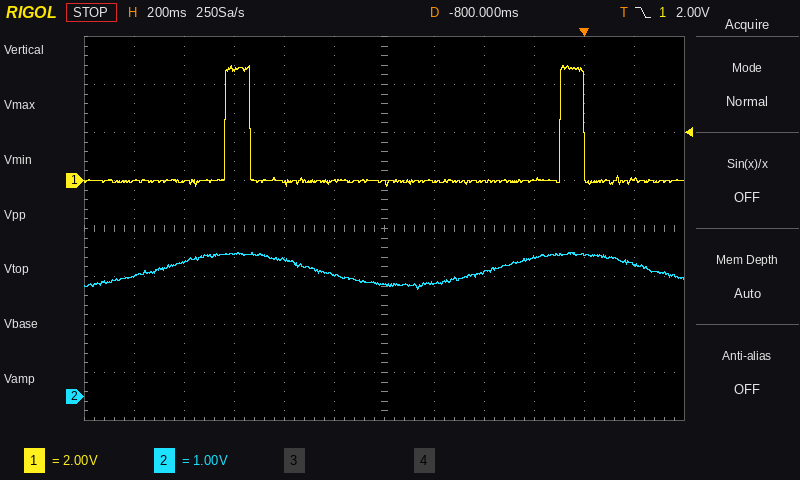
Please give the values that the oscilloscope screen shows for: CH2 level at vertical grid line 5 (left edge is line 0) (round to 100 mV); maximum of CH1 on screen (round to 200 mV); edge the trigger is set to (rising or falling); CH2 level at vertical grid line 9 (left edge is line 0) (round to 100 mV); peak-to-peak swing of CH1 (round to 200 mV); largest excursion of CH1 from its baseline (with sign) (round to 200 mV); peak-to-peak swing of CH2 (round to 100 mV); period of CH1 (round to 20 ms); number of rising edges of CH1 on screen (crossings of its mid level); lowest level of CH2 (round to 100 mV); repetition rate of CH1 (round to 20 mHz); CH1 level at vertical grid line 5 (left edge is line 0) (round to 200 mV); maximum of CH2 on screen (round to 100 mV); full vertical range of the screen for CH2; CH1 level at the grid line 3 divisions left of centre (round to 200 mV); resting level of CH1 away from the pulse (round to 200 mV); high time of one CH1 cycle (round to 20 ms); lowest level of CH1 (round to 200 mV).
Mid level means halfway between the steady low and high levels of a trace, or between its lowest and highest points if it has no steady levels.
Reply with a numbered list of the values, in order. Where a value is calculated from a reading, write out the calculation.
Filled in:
1. 2.5 V
2. 4.8 V
3. falling
4. 2.9 V
5. 4.8 V − (-200 mV) = 5.0 V
6. 4.8 V − (0.0 V) = +4.8 V
7. 3.0 V − (2.2 V) = 800 mV
8. 1.34 s
9. 2
10. 2.2 V
11. 1 / 1.34 s ≈ 746 mHz, so 740 mHz to the nearest 20 mHz
12. 0.0 V
13. 3.0 V
14. 8 V
15. 4.6 V
16. 0.0 V
17. 100 ms
18. -200 mV
